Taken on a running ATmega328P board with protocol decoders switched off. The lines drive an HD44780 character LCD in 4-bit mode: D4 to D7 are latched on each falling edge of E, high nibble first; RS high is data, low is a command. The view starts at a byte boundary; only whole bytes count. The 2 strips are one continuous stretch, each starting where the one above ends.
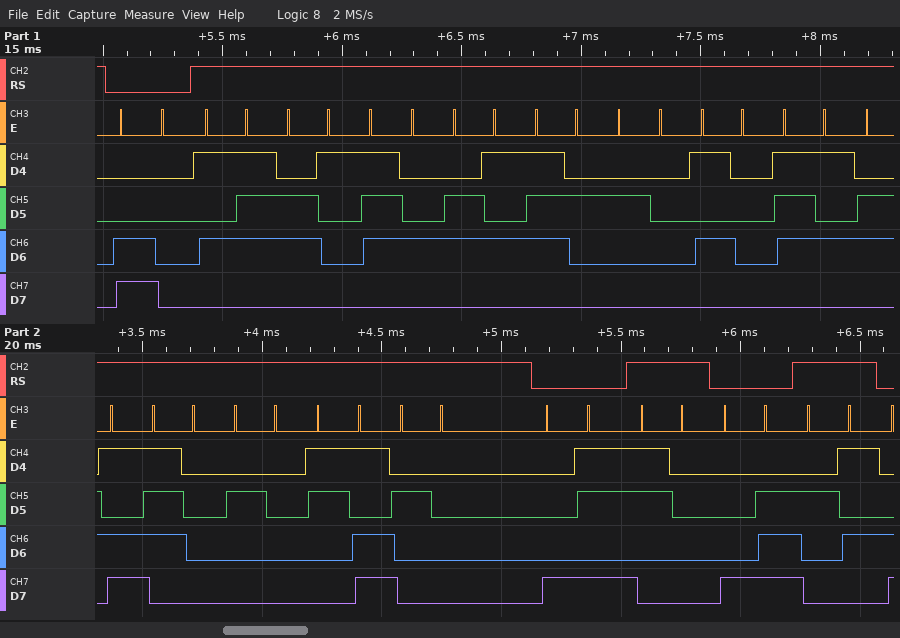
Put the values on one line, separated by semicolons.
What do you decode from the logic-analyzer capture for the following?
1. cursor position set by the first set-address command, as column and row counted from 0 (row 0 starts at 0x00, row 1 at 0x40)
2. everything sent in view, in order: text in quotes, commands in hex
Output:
column 0, row 1; 0xC0 "Water Pump = " 0x8B "0" 0x8E "%"
